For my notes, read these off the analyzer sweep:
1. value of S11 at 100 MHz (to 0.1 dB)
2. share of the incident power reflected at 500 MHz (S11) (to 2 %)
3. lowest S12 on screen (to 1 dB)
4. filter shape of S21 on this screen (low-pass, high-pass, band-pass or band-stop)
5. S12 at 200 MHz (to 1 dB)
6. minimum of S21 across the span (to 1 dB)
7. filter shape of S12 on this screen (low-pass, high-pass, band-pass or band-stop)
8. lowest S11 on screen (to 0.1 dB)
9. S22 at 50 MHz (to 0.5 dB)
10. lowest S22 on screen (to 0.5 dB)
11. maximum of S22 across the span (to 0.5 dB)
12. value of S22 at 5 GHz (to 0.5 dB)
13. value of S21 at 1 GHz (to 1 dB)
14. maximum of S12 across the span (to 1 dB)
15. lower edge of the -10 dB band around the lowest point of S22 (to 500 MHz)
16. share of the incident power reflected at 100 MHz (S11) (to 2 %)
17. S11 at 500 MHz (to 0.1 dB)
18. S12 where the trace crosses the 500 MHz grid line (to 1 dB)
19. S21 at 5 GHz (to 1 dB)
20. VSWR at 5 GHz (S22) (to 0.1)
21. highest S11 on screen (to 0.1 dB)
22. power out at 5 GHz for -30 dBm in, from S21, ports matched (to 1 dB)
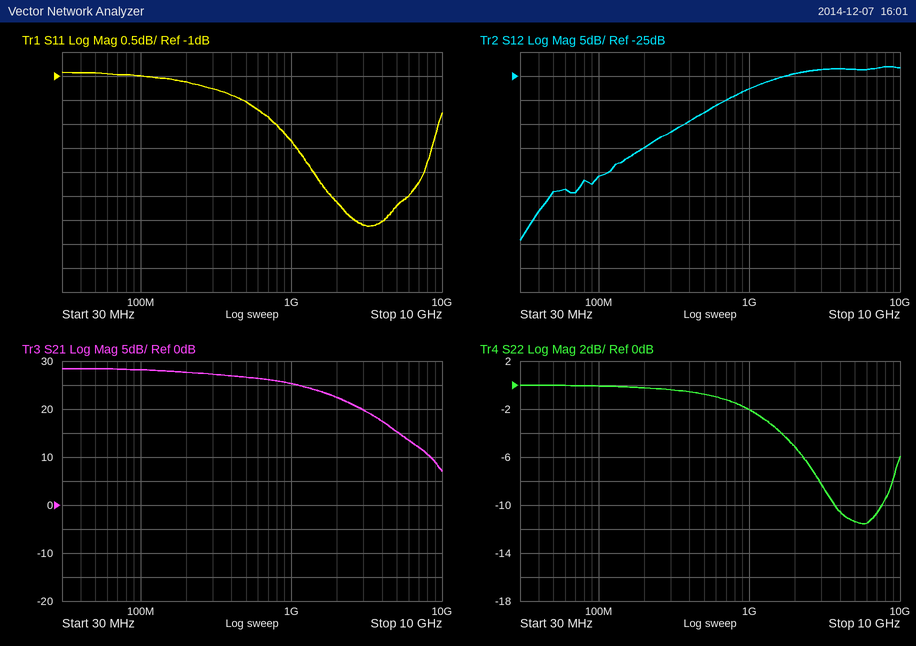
-1.0 dB
70 %
-59 dB
low-pass
-40 dB
7 dB
high-pass
-4.1 dB
0.0 dB
-11.5 dB
0.0 dB
-11.5 dB
25 dB
-23 dB
3.5 GHz
80 %
-1.5 dB
-33 dB
15 dB
1.7
-0.9 dB
-15 dBm
